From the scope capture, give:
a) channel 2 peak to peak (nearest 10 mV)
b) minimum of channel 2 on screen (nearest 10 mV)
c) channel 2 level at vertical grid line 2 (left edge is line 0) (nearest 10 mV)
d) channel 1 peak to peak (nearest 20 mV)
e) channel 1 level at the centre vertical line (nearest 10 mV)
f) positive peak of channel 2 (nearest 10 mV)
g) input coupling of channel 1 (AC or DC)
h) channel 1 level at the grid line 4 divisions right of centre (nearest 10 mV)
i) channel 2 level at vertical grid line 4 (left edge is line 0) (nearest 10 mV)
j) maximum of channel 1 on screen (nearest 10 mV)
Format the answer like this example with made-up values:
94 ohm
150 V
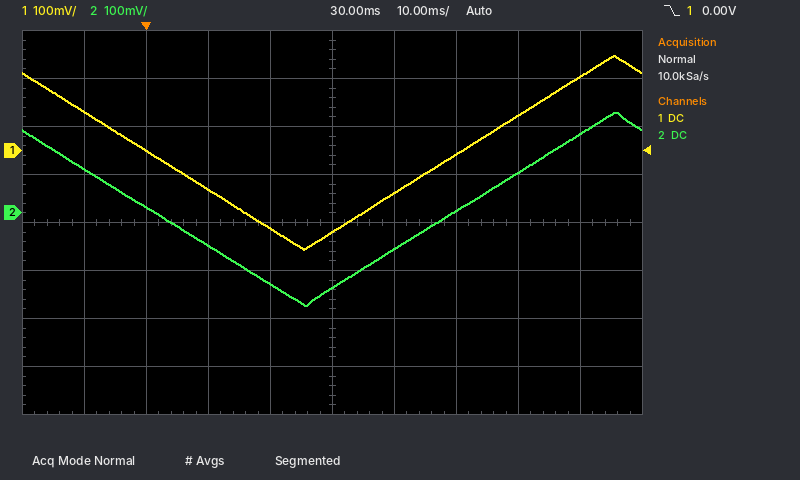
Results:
400 mV
-190 mV
10 mV
400 mV
-170 mV
210 mV
DC
150 mV
-150 mV
200 mV
